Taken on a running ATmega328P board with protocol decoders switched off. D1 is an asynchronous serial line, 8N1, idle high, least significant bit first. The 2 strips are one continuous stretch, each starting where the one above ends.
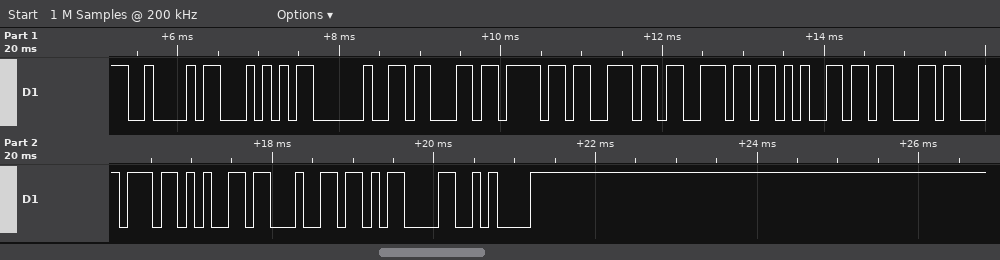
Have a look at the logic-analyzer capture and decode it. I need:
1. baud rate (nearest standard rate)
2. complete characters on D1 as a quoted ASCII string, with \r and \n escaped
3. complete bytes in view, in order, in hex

9600 baud
"BT connected\r\n"
0x42 0x54 0x20 0x63 0x6F 0x6E 0x6E 0x65 0x63 0x74 0x65 0x64 0x0D 0x0A
